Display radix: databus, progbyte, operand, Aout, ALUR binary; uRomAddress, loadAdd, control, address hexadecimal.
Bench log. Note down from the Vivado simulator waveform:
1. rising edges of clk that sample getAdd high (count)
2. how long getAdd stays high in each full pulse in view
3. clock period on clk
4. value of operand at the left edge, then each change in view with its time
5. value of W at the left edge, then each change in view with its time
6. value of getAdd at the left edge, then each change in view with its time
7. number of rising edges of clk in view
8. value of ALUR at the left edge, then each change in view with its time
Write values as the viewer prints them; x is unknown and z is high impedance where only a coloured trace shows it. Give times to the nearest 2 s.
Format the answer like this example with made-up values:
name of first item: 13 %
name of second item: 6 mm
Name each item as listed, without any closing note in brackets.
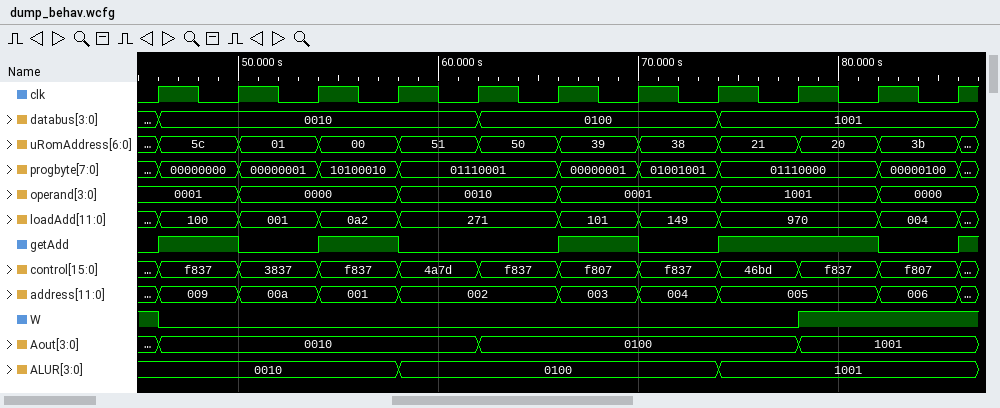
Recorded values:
rising edges of clk that sample getAdd high: 5
how long getAdd stays high in each full pulse in view: 4 s, 4 s, 4 s, 8 s
clock period on clk: 4 s
value of operand at the left edge, then each change in view with its time: 0001, 0000 at 50 s, 0010 at 58 s, 0001 at 66 s, 1001 at 74 s, 0000 at 82 s
value of W at the left edge, then each change in view with its time: 1, 0 at 46 s, 1 at 78 s
value of getAdd at the left edge, then each change in view with its time: 0, 1 at 46 s, 0 at 50 s, 1 at 54 s, 0 at 58 s, 1 at 66 s, 0 at 70 s, 1 at 74 s, 0 at 82 s, 1 at 86 s
number of rising edges of clk in view: 11
value of ALUR at the left edge, then each change in view with its time: 0010, 0100 at 58 s, 1001 at 74 s
